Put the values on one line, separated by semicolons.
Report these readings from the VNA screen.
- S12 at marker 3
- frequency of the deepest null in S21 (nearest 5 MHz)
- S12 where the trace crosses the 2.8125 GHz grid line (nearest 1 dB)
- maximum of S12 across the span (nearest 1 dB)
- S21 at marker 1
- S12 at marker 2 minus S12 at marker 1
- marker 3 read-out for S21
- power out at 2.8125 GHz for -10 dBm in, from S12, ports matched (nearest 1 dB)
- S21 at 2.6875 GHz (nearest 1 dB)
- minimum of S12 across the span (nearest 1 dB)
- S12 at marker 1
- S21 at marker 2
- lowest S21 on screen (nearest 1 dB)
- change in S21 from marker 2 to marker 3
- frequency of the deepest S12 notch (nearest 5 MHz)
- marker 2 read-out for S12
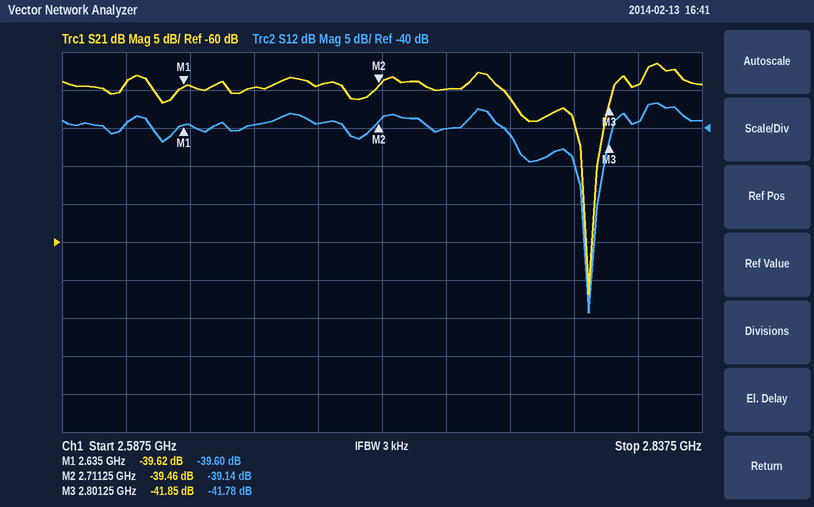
-41.78 dB; 2.795 GHz; -39 dB; -37 dB; -39.62 dB; 0.46 dB; -41.85 dB; -49 dBm; -39 dB; -64 dB; -39.60 dB; -39.46 dB; -67 dB; -2.39 dB; 2.795 GHz; -39.14 dB
